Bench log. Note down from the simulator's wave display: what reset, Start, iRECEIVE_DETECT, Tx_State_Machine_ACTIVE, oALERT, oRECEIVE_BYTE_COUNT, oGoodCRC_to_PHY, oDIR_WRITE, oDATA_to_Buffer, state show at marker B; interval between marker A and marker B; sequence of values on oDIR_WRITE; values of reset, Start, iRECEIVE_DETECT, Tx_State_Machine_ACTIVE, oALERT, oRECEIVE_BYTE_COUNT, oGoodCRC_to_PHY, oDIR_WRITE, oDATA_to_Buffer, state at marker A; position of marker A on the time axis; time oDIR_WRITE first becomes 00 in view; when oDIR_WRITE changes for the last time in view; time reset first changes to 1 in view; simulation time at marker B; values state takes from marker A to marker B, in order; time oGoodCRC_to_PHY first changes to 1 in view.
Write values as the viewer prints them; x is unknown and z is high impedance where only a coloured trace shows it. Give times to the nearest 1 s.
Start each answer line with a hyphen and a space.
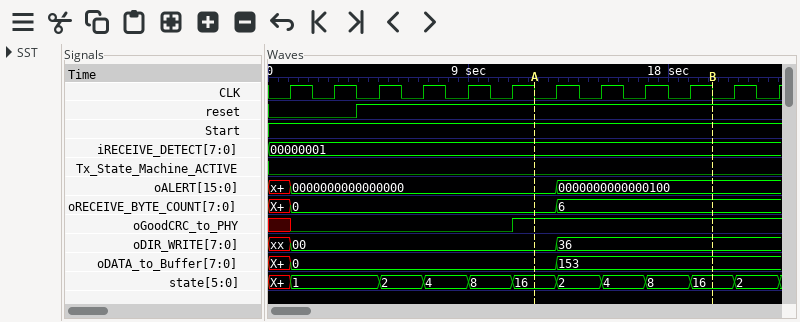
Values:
- reset=1, Start=1, iRECEIVE_DETECT=00000001, Tx_State_Machine_ACTIVE=0, oALERT=0000000000000100, oRECEIVE_BYTE_COUNT=6, oGoodCRC_to_PHY=1, oDIR_WRITE=36, oDATA_to_Buffer=153, state=16
- 8 s
- xx, 00, 36
- reset=1, Start=1, iRECEIVE_DETECT=00000001, Tx_State_Machine_ACTIVE=0, oALERT=0000000000000000, oRECEIVE_BYTE_COUNT=0, oGoodCRC_to_PHY=1, oDIR_WRITE=00, oDATA_to_Buffer=0, state=16
- 12 s
- 1 s
- 13 s
- 4 s
- 20 s
- 16, 2, 4, 8, 16
- 11 s
